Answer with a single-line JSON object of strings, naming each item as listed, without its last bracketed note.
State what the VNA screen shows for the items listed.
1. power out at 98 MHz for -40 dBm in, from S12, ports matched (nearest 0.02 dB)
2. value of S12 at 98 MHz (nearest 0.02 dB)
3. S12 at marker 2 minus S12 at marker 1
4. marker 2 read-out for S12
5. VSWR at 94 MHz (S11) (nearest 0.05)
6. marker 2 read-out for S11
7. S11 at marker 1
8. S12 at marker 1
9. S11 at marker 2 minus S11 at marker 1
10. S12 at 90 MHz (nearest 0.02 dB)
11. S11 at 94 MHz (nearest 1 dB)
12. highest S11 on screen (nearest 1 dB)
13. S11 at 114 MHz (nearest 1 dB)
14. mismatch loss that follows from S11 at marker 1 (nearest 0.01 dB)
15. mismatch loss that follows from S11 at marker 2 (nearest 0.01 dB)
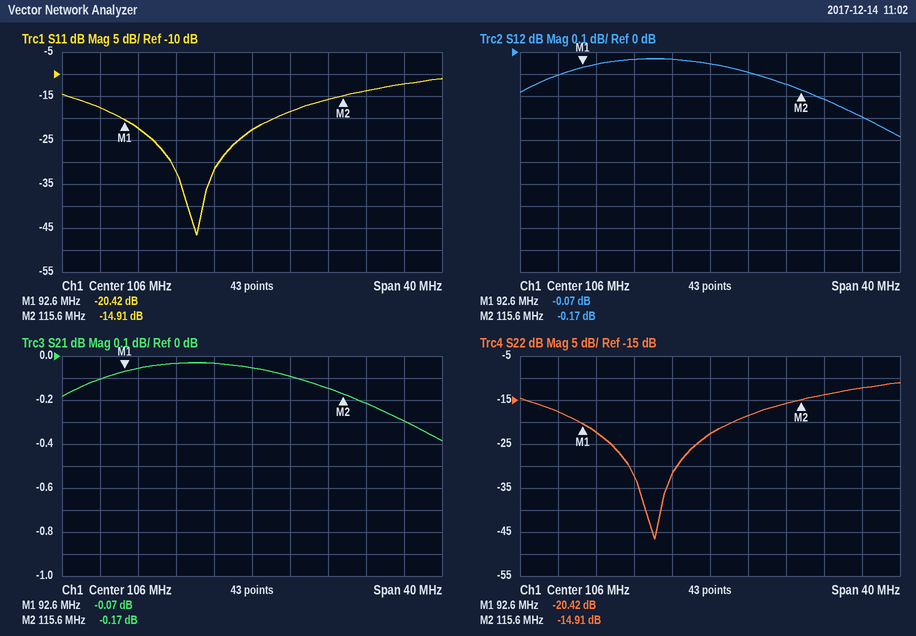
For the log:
{"power out at 98 MHz for -40 dBm in, from S12, ports matched": "-40.04 dBm", "value of S12 at 98 MHz": "-0.04 dB", "S12 at marker 2 minus S12 at marker 1": "-0.10 dB", "marker 2 read-out for S12": "-0.17 dB", "VSWR at 94 MHz (S11)": "1.15", "marker 2 read-out for S11": "-14.91 dB", "S11 at marker 1": "-20.42 dB", "S12 at marker 1": "-0.07 dB", "S11 at marker 2 minus S11 at marker 1": "5.51 dB", "S12 at 90 MHz": "-0.10 dB", "S11 at 94 MHz": "-22 dB", "highest S11 on screen": "-11 dB", "S11 at 114 MHz": "-16 dB", "mismatch loss that follows from S11 at marker 1": "0.04 dB", "mismatch loss that follows from S11 at marker 2": "0.14 dB"}
